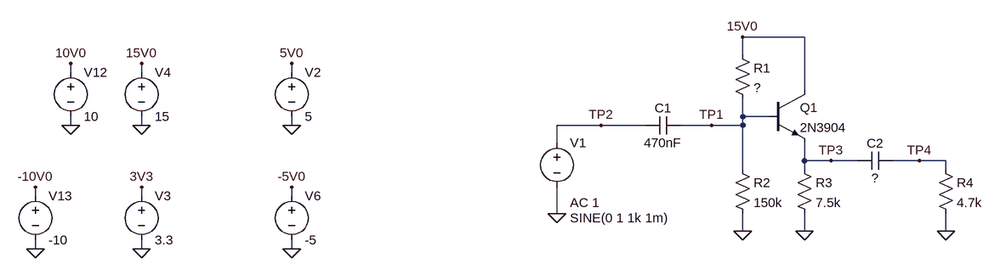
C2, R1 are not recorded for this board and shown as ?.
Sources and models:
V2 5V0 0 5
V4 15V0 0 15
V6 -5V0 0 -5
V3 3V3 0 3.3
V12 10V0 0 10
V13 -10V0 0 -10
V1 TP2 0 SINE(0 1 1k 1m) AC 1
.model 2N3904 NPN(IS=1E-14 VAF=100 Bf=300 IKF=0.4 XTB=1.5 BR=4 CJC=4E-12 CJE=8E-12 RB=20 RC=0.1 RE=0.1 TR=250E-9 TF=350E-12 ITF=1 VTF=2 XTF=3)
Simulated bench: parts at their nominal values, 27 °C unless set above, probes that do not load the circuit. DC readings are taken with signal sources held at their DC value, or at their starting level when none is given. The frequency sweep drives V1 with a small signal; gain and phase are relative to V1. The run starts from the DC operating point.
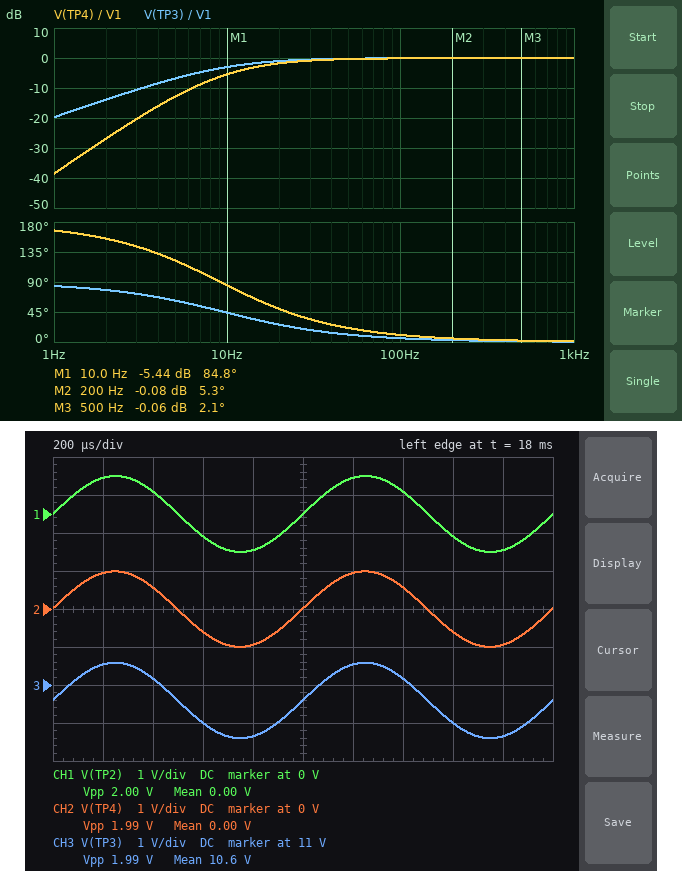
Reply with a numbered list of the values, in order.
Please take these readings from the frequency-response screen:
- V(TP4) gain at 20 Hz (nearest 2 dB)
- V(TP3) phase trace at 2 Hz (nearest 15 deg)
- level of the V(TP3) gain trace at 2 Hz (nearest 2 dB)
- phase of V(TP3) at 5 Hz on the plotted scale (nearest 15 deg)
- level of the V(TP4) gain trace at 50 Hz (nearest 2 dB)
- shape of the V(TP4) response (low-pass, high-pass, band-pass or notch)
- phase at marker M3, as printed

1. -2 dB
2. 75 deg
3. -14 dB
4. 60 deg
5. 0 dB
6. high-pass
7. 2.1 deg
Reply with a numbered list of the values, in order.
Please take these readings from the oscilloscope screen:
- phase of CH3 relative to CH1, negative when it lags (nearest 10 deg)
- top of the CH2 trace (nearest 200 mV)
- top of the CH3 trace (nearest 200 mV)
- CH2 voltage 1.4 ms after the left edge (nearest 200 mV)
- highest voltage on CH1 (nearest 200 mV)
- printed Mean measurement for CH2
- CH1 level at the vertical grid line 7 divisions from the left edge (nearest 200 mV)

1. 0 deg
2. 1.0 V
3. 11.6 V
4. 600 mV
5. 1.0 V
6. 0.00 V
7. 600 mV
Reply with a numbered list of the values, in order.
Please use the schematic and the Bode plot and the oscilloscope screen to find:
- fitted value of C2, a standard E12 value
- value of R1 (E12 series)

1. 3.9 µF
2. 47 kΩ
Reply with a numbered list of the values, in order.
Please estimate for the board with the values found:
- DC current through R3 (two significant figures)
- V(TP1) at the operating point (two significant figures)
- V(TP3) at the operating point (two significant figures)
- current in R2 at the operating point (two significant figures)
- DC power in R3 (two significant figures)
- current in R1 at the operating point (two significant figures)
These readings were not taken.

1. 1.4 mA
2. 11 V
3. 11 V
4. 75 µA
5. 15 mW
6. 80 µA
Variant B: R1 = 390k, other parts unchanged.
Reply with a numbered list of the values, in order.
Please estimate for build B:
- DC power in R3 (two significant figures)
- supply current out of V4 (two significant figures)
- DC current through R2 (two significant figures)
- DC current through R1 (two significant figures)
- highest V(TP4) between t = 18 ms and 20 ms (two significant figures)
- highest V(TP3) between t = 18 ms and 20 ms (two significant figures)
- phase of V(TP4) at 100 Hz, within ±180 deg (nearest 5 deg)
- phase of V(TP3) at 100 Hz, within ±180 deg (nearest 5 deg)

1. 1.5 mW
2. 480 µA
3. 27 µA
4. 28 µA
5. 980 mV
6. 4.4 V
7. 5 deg
8. 0 deg
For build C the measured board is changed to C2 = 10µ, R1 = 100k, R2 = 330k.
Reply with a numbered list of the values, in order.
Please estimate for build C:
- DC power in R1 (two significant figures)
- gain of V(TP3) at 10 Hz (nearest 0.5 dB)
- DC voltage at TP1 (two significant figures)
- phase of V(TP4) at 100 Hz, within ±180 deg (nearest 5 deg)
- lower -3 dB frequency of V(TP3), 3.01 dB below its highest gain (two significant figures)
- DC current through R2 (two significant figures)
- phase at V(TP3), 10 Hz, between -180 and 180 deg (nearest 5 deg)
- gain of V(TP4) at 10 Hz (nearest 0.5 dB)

1. 150 µW
2. -1.0 dB
3. 11 V
4. 5 deg
5. 4.8 Hz
6. 34 µA
7. 25 deg
8. -1.5 dB
